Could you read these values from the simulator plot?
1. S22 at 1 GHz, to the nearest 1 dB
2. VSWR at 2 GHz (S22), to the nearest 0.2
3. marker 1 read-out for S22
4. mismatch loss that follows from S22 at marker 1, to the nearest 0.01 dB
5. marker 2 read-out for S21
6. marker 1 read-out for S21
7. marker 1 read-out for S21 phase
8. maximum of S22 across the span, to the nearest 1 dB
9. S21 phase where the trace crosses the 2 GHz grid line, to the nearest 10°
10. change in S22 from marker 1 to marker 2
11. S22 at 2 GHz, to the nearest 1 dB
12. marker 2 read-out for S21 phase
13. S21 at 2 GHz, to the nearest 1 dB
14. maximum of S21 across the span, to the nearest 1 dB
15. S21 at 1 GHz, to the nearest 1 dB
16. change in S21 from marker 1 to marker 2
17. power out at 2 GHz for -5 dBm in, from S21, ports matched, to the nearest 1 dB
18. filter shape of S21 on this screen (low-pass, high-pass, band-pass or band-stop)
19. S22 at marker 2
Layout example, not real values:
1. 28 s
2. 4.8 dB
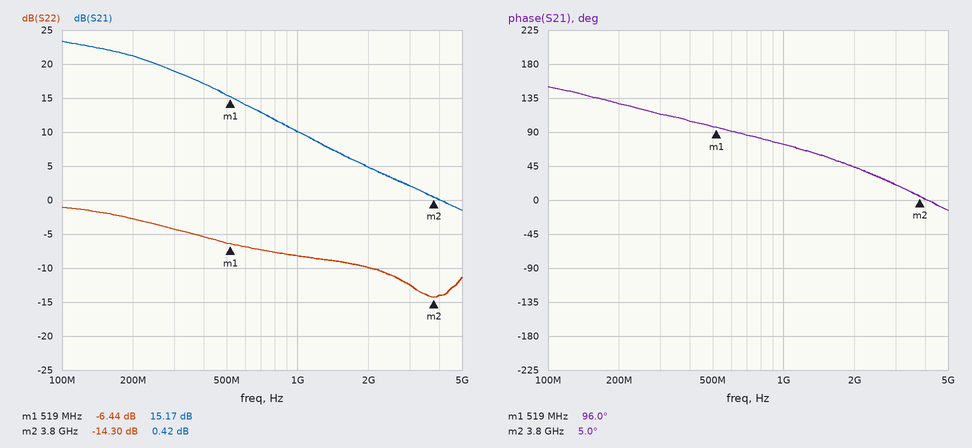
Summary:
1. -8 dB
2. 2.0
3. -6.44 dB
4. 1.12 dB
5. 0.42 dB
6. 15.17 dB
7. 96.0°
8. -1 dB
9. 40°
10. -7.86 dB
11. -10 dB
12. 5.0°
13. 5 dB
14. 23 dB
15. 10 dB
16. -14.75 dB
17. 0 dBm
18. low-pass
19. -14.30 dB
